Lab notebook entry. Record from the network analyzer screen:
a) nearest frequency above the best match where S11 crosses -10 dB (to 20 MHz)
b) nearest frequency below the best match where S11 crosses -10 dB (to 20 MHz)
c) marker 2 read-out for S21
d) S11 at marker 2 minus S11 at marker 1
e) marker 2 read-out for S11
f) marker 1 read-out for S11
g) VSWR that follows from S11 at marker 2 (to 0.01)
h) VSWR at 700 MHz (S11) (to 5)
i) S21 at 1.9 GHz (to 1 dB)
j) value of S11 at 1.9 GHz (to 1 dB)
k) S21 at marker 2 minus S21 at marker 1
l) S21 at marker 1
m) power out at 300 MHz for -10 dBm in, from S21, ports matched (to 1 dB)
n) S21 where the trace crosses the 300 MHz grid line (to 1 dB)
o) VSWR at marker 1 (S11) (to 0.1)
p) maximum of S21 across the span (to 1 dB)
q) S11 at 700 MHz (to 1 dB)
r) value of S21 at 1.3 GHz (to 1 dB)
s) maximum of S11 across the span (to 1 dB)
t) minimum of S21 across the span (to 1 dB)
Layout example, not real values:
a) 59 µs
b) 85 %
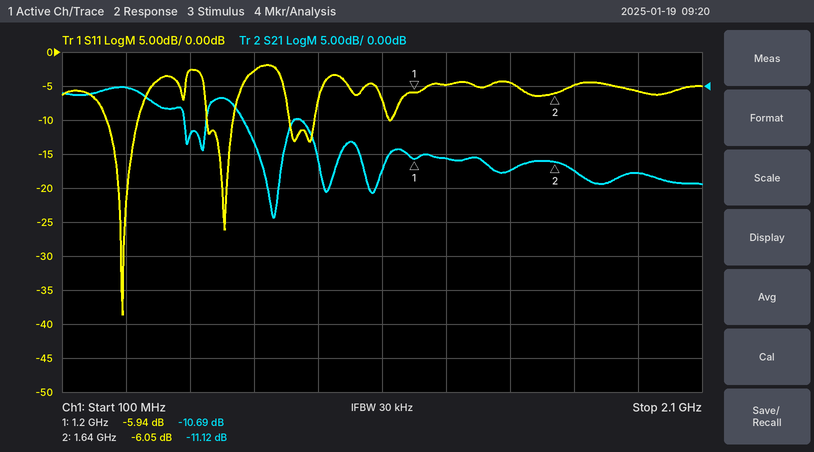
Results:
a) 340 MHz
b) 240 MHz
c) -11.12 dB
d) -0.11 dB
e) -6.05 dB
f) -5.94 dB
g) 2.99
h) 5
i) -13 dB
j) -6 dB
k) -0.43 dB
l) -10.69 dB
m) -10 dBm
n) 0 dB
o) 3.0
p) 0 dB
q) -3 dB
r) -11 dB
s) -2 dB
t) -19 dB
